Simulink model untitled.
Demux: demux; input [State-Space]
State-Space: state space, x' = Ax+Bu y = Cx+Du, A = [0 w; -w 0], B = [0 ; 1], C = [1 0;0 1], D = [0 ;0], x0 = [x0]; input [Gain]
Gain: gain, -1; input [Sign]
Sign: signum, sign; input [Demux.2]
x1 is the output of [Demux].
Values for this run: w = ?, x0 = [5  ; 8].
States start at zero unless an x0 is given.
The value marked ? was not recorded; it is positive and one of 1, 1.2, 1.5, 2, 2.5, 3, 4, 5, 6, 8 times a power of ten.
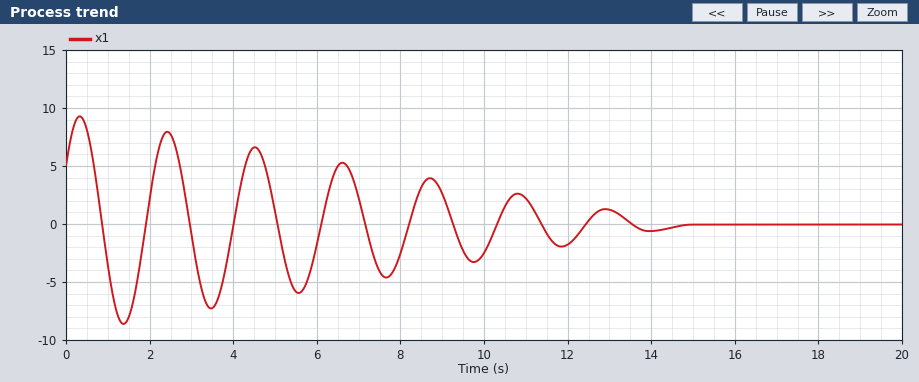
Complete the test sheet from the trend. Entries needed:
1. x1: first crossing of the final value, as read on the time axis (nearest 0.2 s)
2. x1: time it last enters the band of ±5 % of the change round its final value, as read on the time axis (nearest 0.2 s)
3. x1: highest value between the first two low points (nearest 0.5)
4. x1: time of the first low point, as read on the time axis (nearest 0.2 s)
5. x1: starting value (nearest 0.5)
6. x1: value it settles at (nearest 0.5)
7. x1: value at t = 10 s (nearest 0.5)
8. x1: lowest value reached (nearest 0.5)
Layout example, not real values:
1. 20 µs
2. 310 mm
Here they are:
1. 0.8 s
2. 14.6 s
3. 8.0
4. 1.4 s
5. 5.0
6. 0.0
7. -2.5
8. -8.5
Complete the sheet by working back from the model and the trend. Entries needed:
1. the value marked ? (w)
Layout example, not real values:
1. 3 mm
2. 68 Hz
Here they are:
1. 3
